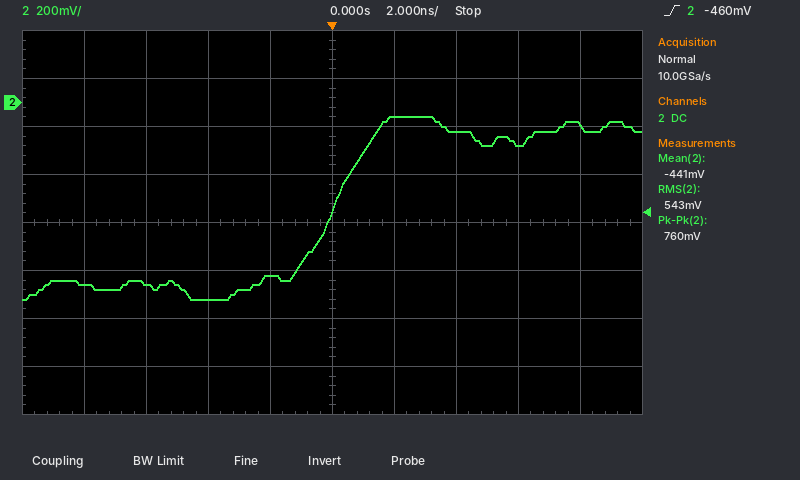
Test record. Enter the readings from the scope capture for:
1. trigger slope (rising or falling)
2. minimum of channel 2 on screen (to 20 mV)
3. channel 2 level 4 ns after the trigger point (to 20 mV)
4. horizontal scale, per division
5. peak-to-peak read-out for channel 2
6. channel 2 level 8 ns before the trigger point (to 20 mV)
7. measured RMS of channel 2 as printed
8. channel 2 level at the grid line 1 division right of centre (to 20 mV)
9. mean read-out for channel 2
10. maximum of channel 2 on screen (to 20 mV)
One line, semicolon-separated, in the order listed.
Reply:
rising; -820 mV; -120 mV; 2 ns; 760 mV; -760 mV; 543 mV; -60 mV; -441 mV; -60 mV
